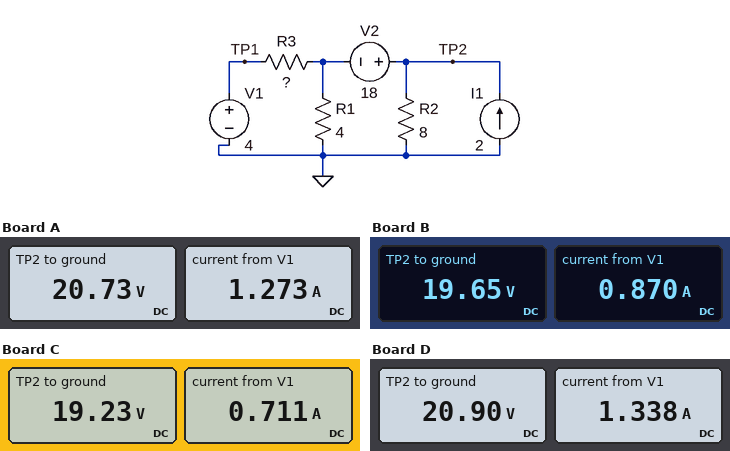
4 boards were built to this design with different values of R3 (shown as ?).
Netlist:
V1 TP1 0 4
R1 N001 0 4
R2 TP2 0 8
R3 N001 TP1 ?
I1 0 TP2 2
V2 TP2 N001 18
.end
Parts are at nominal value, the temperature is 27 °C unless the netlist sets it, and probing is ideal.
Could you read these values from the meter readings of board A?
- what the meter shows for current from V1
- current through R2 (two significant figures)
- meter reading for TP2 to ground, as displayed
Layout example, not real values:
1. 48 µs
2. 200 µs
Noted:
1. 1.273 A
2. 2.6 A
3. 20.73 V
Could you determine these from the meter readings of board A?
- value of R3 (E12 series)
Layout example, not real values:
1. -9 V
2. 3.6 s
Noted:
1. 1 Ω
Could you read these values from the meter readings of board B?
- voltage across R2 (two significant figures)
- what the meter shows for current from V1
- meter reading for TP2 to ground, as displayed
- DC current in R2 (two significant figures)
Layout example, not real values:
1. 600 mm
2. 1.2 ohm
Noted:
1. 20 V
2. 0.870 A
3. 19.65 V
4. 2.5 A
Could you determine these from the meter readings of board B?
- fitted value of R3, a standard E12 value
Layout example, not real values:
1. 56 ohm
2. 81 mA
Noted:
1. 2.7 Ω
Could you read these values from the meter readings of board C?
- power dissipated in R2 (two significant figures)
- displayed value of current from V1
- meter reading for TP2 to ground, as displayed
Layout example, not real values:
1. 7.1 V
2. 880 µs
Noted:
1. 46 W
2. 0.711 A
3. 19.23 V
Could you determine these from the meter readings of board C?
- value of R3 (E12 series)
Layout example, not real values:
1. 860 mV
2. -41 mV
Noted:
1. 3.9 Ω
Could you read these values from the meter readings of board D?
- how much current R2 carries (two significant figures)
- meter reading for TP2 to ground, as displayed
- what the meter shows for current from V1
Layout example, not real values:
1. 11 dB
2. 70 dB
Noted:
1. 2.6 A
2. 20.90 V
3. 1.338 A
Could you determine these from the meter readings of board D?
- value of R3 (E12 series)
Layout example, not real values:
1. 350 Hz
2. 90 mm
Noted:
1. 0.82 Ω
